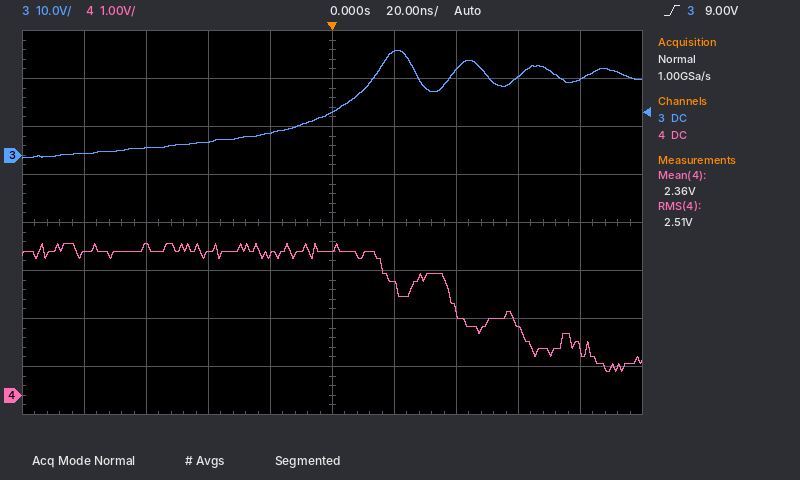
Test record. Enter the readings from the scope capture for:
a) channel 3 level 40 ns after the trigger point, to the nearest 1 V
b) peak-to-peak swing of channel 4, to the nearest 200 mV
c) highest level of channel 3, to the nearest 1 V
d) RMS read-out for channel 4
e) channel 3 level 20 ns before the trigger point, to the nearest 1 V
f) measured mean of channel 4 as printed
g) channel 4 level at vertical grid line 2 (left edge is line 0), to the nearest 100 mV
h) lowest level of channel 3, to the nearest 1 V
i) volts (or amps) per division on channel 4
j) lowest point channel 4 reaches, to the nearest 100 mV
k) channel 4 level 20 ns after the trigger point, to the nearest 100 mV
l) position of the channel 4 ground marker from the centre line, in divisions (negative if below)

18 V
2.6 V
22 V
2.51 V
5 V
2.36 V
3.1 V
-1 V
1 V
500 mV
2.3 V
-3.6 div
